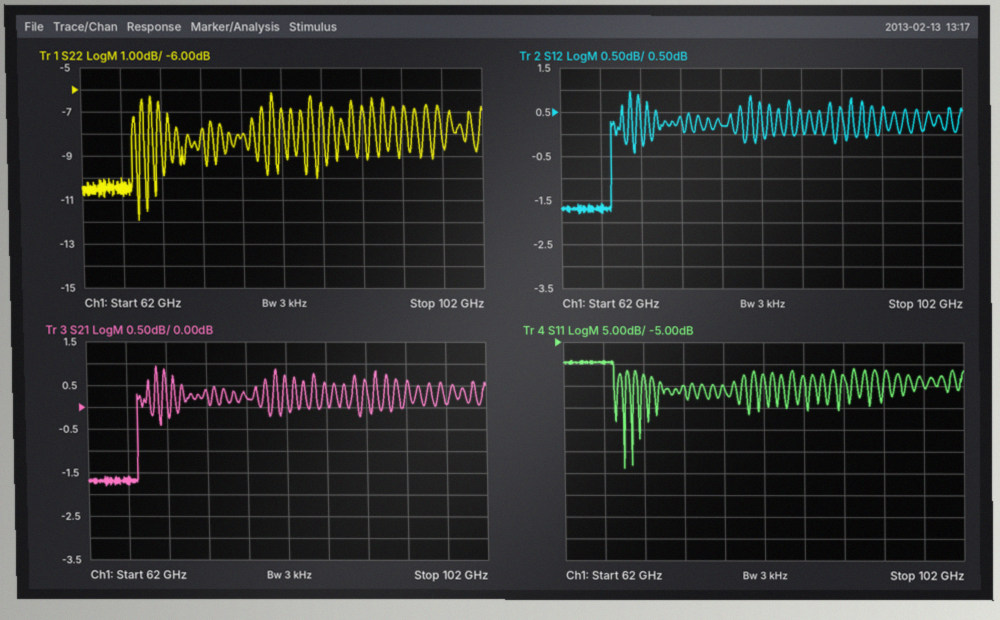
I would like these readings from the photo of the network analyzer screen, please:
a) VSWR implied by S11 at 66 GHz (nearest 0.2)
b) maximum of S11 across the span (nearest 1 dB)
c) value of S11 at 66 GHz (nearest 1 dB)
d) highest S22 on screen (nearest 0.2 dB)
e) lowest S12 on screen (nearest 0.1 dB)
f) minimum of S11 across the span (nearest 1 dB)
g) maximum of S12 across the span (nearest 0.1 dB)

2.0
-9 dB
-10 dB
-6.2 dB
-1.8 dB
-34 dB
1.0 dB
